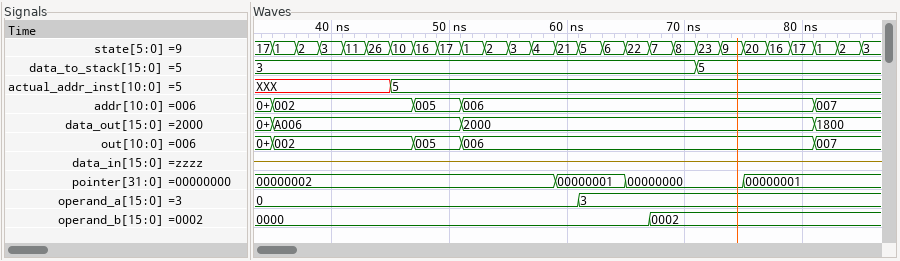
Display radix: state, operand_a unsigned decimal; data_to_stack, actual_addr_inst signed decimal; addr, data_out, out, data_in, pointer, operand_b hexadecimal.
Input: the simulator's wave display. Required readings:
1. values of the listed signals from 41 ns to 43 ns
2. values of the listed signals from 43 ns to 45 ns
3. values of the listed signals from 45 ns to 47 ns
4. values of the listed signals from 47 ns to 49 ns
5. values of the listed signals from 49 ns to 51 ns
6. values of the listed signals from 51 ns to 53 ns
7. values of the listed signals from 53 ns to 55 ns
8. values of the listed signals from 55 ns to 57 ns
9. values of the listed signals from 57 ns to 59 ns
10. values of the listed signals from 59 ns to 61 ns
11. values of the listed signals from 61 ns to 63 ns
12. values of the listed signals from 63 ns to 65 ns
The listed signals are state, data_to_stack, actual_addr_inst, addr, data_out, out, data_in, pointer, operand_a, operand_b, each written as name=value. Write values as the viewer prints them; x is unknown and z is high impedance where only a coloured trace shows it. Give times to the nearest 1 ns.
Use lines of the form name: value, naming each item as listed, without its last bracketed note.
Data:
values of the listed signals from 41 ns to 43 ns: state=11, data_to_stack=3, actual_addr_inst=XXX, addr=002, data_out=A006, out=002, data_in=z, pointer=00000002, operand_a=0, operand_b=0000
values of the listed signals from 43 ns to 45 ns: state=26, data_to_stack=3, actual_addr_inst=XXX, addr=002, data_out=A006, out=002, data_in=z, pointer=00000002, operand_a=0, operand_b=0000
values of the listed signals from 45 ns to 47 ns: state=10, data_to_stack=3, actual_addr_inst=5, addr=002, data_out=A006, out=002, data_in=z, pointer=00000002, operand_a=0, operand_b=0000
values of the listed signals from 47 ns to 49 ns: state=16, data_to_stack=3, actual_addr_inst=5, addr=005, data_out=A006, out=005, data_in=z, pointer=00000002, operand_a=0, operand_b=0000
values of the listed signals from 49 ns to 51 ns: state=17, data_to_stack=3, actual_addr_inst=5, addr=005, data_out=A006, out=005, data_in=z, pointer=00000002, operand_a=0, operand_b=0000
values of the listed signals from 51 ns to 53 ns: state=1, data_to_stack=3, actual_addr_inst=5, addr=006, data_out=2000, out=006, data_in=z, pointer=00000002, operand_a=0, operand_b=0000
values of the listed signals from 53 ns to 55 ns: state=2, data_to_stack=3, actual_addr_inst=5, addr=006, data_out=2000, out=006, data_in=z, pointer=00000002, operand_a=0, operand_b=0000
values of the listed signals from 55 ns to 57 ns: state=3, data_to_stack=3, actual_addr_inst=5, addr=006, data_out=2000, out=006, data_in=z, pointer=00000002, operand_a=0, operand_b=0000
values of the listed signals from 57 ns to 59 ns: state=4, data_to_stack=3, actual_addr_inst=5, addr=006, data_out=2000, out=006, data_in=z, pointer=00000002, operand_a=0, operand_b=0000
values of the listed signals from 59 ns to 61 ns: state=21, data_to_stack=3, actual_addr_inst=5, addr=006, data_out=2000, out=006, data_in=z, pointer=00000001, operand_a=0, operand_b=0000
values of the listed signals from 61 ns to 63 ns: state=5, data_to_stack=3, actual_addr_inst=5, addr=006, data_out=2000, out=006, data_in=z, pointer=00000001, operand_a=3, operand_b=0000
values of the listed signals from 63 ns to 65 ns: state=6, data_to_stack=3, actual_addr_inst=5, addr=006, data_out=2000, out=006, data_in=z, pointer=00000001, operand_a=3, operand_b=0000
